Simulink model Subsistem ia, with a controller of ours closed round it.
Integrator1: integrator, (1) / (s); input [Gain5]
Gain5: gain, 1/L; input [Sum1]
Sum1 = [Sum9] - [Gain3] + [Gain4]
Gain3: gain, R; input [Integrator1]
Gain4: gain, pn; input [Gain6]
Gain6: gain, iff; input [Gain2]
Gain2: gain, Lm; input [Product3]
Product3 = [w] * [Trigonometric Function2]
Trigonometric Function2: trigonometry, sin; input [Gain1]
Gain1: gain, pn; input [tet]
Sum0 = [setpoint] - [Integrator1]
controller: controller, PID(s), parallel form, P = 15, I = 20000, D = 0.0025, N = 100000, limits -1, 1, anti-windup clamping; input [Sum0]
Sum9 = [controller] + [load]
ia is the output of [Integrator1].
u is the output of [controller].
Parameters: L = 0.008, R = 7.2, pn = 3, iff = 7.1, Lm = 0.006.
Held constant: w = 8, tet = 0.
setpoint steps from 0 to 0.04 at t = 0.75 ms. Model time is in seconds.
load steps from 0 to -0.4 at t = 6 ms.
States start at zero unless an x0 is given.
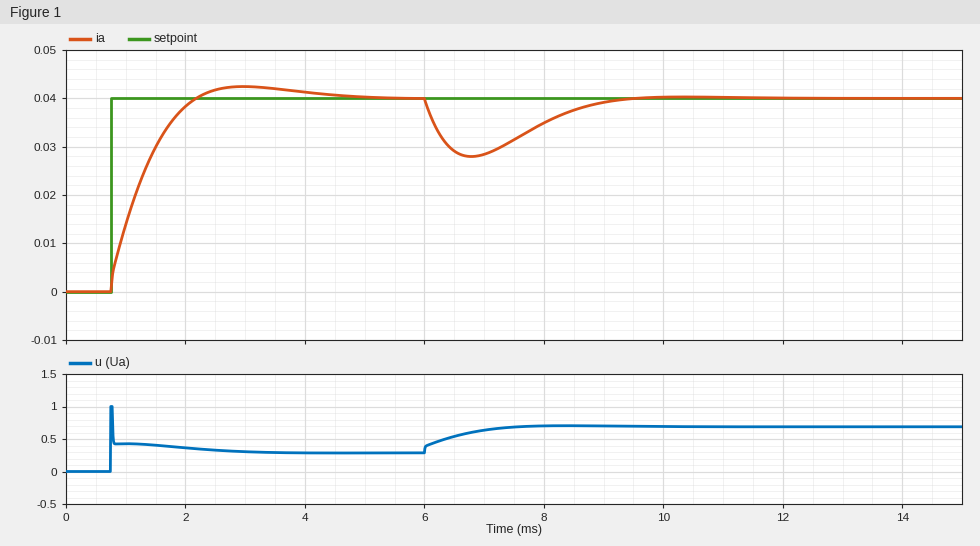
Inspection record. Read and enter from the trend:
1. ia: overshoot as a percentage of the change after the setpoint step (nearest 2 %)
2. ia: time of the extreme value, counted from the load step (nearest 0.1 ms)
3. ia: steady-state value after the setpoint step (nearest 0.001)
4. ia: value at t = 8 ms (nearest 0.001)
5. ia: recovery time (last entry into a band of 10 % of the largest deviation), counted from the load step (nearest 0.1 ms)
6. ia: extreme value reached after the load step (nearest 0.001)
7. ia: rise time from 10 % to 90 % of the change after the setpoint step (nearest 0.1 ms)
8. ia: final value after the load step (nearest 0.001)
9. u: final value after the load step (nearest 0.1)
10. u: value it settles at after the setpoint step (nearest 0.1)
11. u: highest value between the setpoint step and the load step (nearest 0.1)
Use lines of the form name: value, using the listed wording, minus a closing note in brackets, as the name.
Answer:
ia: overshoot as a percentage of the change after the setpoint step: 6 %
ia: time of the extreme value, counted from the load step: 0.8 ms
ia: steady-state value after the setpoint step: 0.040
ia: value at t = 8 ms: 0.035
ia: recovery time (last entry into a band of 10 % of the largest deviation), counted from the load step: 2.9 ms
ia: extreme value reached after the load step: 0.028
ia: rise time from 10 % to 90 % of the change after the setpoint step: 1.0 ms
ia: final value after the load step: 0.040
u: final value after the load step: 0.7
u: value it settles at after the setpoint step: 0.3
u: highest value between the setpoint step and the load step: 1.0
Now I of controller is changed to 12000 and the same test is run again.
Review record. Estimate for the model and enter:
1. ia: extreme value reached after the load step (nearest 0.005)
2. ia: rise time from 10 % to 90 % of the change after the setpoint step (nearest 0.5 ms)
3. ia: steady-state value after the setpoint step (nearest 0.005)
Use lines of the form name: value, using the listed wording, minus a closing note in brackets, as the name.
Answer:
ia: extreme value reached after the load step: 0.025
ia: rise time from 10 % to 90 % of the change after the setpoint step: 1.5 ms
ia: steady-state value after the setpoint step: 0.040
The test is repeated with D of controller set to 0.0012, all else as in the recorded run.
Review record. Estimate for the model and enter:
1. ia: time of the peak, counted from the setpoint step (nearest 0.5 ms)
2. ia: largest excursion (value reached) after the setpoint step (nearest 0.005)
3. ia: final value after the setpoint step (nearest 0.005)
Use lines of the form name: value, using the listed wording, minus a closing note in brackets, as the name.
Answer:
ia: time of the peak, counted from the setpoint step: 2.0 ms
ia: largest excursion (value reached) after the setpoint step: 0.040
ia: final value after the setpoint step: 0.040
